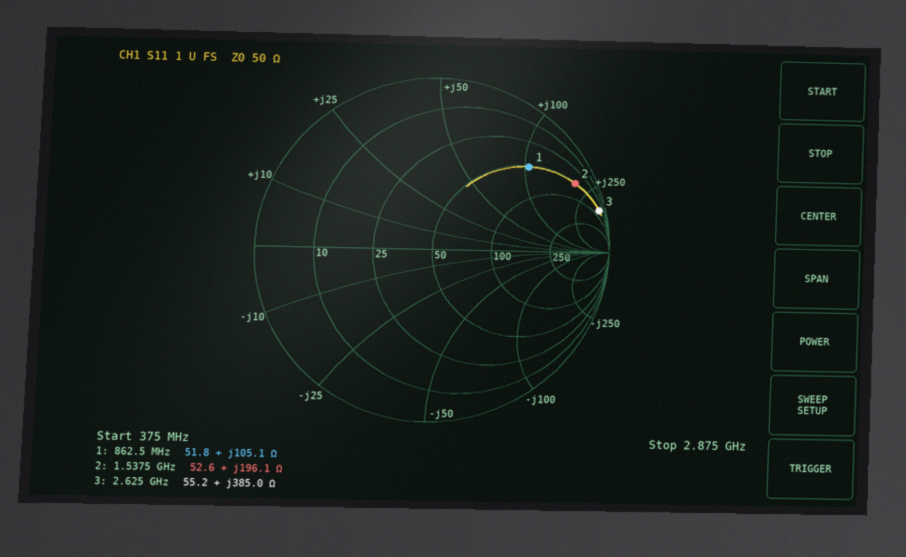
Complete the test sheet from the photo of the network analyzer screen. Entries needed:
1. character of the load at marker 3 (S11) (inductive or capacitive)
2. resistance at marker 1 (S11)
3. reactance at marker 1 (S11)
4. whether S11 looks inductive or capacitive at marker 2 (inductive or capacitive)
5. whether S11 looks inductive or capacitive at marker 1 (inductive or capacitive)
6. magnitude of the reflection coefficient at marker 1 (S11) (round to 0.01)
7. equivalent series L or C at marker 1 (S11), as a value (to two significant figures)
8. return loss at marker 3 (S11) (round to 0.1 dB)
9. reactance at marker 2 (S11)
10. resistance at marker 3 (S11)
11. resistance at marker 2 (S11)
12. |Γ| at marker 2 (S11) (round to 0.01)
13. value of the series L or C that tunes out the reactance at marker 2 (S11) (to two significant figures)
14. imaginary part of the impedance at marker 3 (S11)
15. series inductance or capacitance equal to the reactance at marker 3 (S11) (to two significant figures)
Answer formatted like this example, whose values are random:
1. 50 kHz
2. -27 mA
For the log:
1. inductive
2. 51.8 Ω
3. +105.1 Ω
4. inductive
5. inductive
6. 0.72
7. 19 nH
8. 0.3 dB
9. +196.1 Ω
10. 55.2 Ω
11. 52.6 Ω
12. 0.89
13. 530 fF
14. +385.0 Ω
15. 23 nH
